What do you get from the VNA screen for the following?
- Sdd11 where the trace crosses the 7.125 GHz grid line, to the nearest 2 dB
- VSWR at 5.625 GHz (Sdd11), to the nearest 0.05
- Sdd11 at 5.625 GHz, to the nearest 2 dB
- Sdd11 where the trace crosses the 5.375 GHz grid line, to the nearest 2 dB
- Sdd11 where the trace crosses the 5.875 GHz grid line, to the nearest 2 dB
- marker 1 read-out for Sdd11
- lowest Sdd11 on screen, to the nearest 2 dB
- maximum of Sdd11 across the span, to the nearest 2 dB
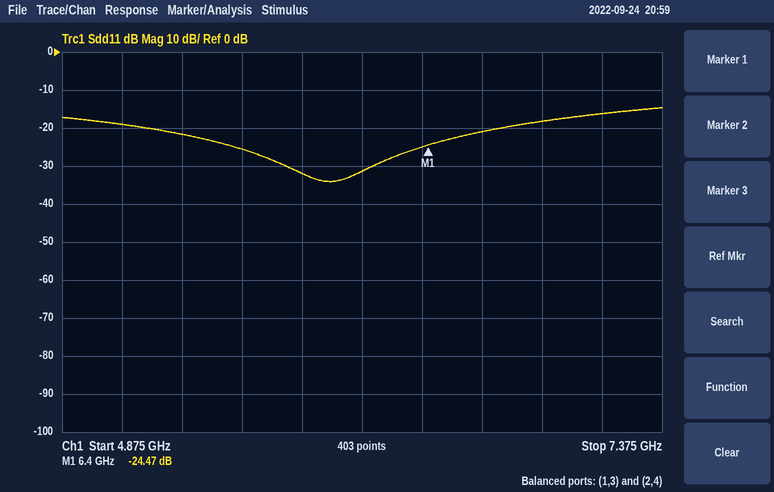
-16 dB
1.10
-26 dB
-22 dB
-32 dB
-24.47 dB
-34 dB
-14 dB
